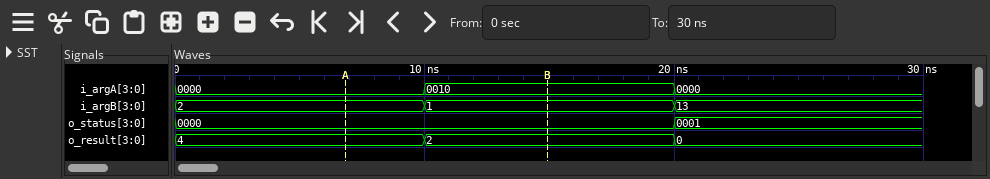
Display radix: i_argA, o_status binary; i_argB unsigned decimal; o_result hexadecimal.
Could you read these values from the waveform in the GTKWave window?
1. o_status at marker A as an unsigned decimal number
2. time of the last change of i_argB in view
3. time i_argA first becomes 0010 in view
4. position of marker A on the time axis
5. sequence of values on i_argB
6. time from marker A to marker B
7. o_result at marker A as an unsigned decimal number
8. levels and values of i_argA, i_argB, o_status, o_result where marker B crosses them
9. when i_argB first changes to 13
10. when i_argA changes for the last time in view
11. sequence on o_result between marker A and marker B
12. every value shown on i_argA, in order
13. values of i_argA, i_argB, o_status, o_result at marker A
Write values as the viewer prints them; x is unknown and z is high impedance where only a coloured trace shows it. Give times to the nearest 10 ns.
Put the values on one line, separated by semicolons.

0; 20 ns; 10 ns; 10 ns; 2, 1, 13; 10 ns; 4; i_argA=0010, i_argB=1, o_status=0000, o_result=2; 20 ns; 20 ns; 4, 2; 0000, 0010, 0000; i_argA=0000, i_argB=2, o_status=0000, o_result=4
